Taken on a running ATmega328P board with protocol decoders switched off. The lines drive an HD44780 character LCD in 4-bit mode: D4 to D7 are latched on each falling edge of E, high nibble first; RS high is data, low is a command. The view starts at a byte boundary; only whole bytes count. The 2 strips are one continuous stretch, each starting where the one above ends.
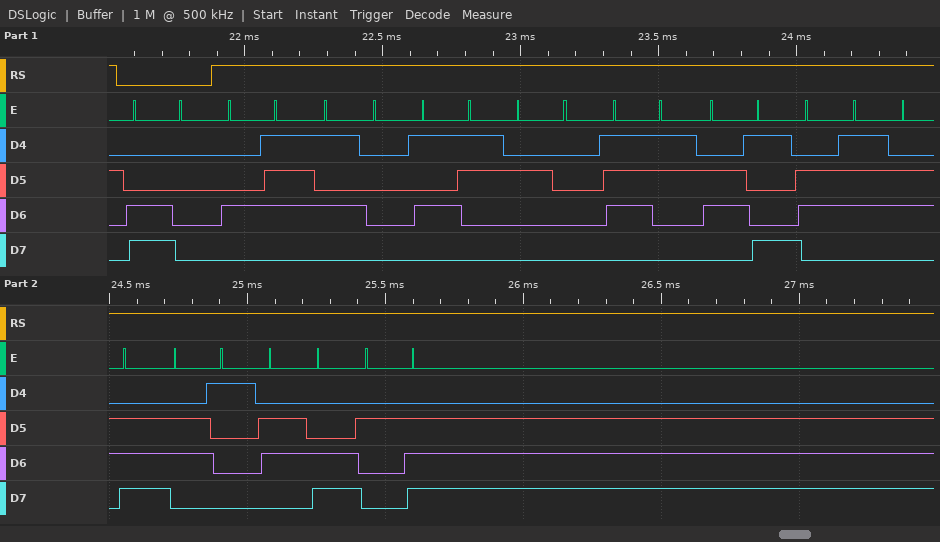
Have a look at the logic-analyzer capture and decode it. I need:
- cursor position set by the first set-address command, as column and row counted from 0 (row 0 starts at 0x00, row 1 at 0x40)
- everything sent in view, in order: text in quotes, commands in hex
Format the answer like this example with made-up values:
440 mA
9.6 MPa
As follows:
column 0, row 1
0xC0 "GPS signal."
